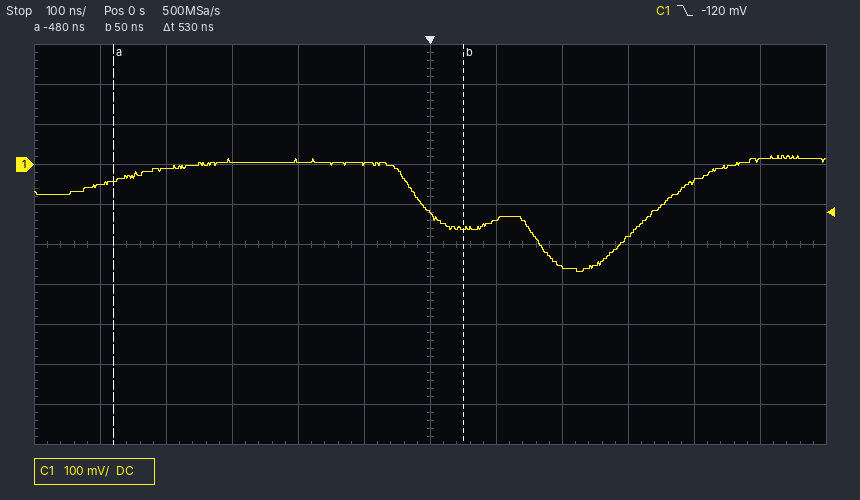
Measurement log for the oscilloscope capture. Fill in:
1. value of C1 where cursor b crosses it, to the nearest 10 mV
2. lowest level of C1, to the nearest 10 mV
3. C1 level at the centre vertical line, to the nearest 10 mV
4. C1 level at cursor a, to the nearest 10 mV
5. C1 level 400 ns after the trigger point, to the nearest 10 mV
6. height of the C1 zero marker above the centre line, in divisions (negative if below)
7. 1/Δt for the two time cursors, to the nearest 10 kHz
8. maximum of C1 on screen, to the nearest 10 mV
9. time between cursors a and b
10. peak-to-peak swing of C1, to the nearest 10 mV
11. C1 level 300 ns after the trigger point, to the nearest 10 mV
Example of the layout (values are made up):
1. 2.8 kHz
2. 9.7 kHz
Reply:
1. -160 mV
2. -270 mV
3. -120 mV
4. -40 mV
5. -40 mV
6. +2.0 div
7. 1.89 MHz
8. 20 mV
9. 530 ns
10. 290 mV
11. -180 mV
